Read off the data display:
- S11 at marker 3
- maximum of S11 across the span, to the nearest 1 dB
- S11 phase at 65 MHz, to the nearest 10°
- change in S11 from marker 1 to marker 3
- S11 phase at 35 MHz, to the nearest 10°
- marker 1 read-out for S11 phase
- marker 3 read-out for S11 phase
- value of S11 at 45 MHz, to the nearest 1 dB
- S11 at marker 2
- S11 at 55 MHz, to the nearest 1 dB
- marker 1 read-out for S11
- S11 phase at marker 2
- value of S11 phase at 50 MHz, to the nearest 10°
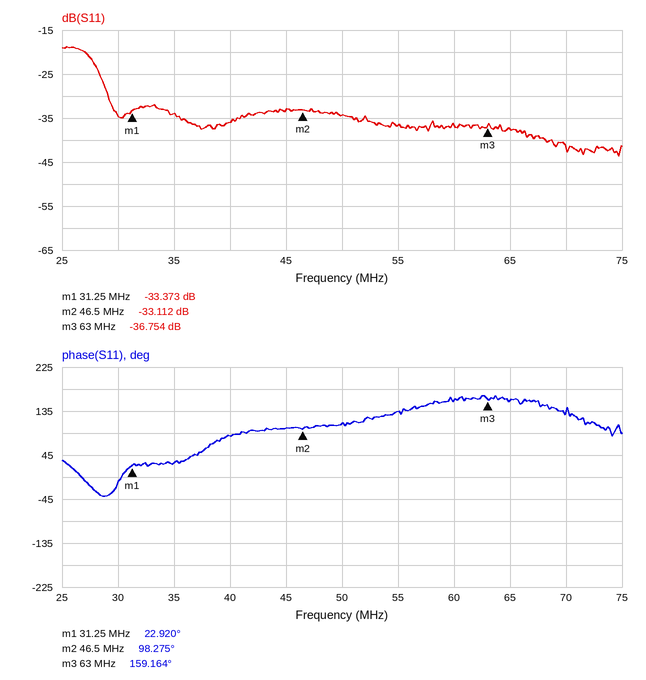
-36.754 dB
-19 dB
160°
-3.381 dB
30°
22.920°
159.164°
-33 dB
-33.112 dB
-37 dB
-33.373 dB
98.275°
110°
